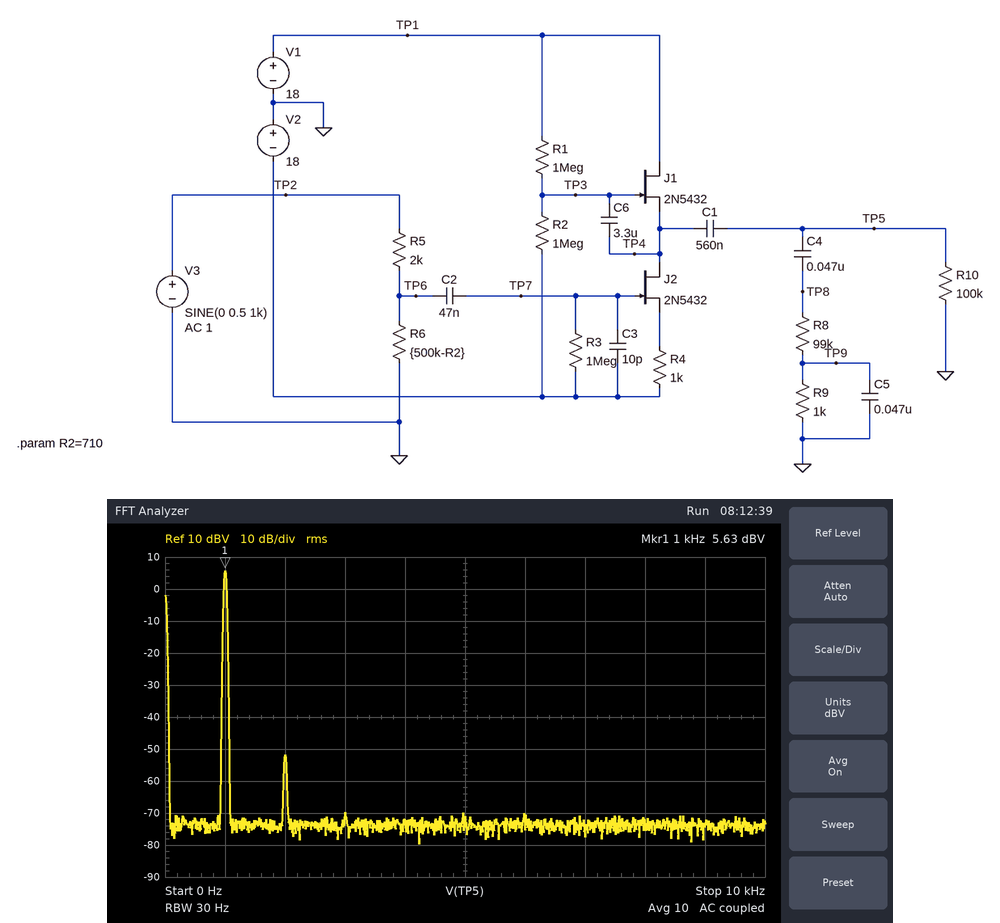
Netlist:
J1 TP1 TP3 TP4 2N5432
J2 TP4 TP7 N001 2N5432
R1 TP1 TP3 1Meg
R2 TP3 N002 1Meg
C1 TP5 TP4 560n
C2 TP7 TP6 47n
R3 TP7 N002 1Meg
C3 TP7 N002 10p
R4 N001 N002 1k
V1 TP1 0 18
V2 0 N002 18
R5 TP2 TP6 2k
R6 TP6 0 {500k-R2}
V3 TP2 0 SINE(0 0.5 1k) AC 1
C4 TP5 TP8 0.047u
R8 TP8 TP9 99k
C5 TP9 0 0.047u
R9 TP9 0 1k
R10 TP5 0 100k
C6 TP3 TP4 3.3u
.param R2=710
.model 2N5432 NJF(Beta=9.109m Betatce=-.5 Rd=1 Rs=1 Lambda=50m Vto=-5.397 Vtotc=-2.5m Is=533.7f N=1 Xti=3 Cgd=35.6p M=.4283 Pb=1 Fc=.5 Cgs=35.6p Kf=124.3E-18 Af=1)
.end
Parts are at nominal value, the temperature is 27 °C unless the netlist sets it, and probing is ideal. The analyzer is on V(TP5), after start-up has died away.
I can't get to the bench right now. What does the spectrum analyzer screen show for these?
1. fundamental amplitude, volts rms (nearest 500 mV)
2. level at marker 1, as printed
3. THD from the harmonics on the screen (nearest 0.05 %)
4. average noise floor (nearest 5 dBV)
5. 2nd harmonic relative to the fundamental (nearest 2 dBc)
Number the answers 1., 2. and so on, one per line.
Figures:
1. 2.0 V
2. 5.63 dBV
3. 0.15 %
4. -75 dBV
5. -58 dBc
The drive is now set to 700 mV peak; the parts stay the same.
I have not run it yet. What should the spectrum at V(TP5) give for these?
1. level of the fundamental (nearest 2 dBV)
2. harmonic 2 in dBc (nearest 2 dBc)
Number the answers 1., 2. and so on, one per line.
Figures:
1. 8 dBV
2. -54 dBc
